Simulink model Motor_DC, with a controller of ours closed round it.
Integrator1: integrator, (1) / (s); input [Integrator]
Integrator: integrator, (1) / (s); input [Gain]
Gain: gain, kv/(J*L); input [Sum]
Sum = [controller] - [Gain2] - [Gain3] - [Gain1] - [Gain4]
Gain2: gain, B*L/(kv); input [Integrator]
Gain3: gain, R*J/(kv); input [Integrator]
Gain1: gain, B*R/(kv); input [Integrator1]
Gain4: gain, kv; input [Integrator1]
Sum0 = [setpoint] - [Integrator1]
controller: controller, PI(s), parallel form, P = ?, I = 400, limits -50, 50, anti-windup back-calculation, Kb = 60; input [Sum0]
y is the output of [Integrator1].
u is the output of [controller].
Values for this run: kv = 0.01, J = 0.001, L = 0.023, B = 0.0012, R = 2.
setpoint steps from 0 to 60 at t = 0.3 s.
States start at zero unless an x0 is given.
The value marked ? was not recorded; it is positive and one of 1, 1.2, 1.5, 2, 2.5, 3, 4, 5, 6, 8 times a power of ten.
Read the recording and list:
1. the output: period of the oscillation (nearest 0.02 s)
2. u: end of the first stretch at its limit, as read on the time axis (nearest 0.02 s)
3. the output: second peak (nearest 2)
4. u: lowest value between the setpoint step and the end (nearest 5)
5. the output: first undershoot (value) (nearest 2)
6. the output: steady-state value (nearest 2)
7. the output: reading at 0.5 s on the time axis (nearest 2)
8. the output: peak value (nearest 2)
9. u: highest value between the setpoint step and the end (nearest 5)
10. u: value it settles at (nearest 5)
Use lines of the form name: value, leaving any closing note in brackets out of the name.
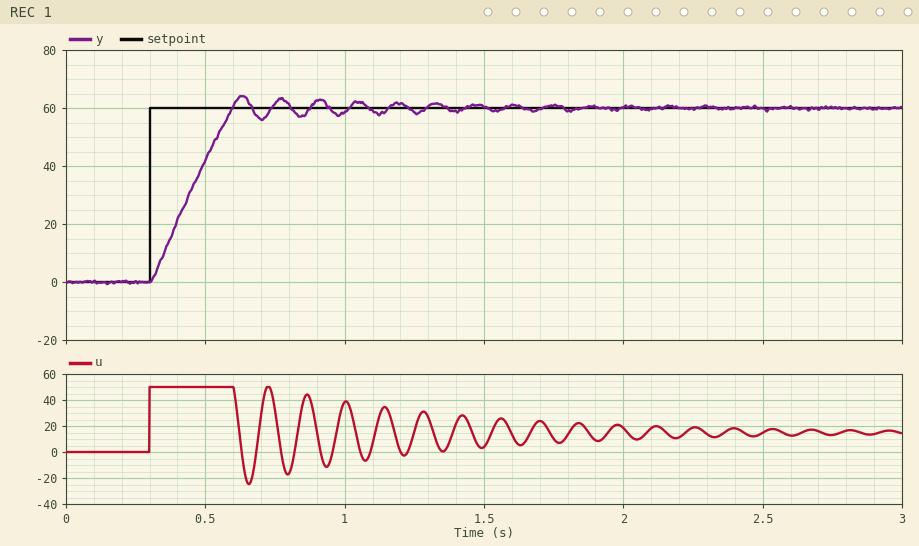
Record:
the output: period of the oscillation: 0.14 s
u: end of the first stretch at its limit, as read on the time axis: 0.60 s
the output: second peak: 64
u: lowest value between the setpoint step and the end: -25
the output: first undershoot (value): 56
the output: steady-state value: 60
the output: reading at 0.5 s on the time axis: 42
the output: peak value: 64
u: highest value between the setpoint step and the end: 50
u: value it settles at: 15
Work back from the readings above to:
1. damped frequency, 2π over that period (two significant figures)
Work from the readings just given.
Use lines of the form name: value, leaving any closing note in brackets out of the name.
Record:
damped frequency, 2π over that period: 45 rad/s
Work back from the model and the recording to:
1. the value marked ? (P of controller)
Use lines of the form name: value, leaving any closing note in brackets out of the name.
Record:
the value marked ?: 5
